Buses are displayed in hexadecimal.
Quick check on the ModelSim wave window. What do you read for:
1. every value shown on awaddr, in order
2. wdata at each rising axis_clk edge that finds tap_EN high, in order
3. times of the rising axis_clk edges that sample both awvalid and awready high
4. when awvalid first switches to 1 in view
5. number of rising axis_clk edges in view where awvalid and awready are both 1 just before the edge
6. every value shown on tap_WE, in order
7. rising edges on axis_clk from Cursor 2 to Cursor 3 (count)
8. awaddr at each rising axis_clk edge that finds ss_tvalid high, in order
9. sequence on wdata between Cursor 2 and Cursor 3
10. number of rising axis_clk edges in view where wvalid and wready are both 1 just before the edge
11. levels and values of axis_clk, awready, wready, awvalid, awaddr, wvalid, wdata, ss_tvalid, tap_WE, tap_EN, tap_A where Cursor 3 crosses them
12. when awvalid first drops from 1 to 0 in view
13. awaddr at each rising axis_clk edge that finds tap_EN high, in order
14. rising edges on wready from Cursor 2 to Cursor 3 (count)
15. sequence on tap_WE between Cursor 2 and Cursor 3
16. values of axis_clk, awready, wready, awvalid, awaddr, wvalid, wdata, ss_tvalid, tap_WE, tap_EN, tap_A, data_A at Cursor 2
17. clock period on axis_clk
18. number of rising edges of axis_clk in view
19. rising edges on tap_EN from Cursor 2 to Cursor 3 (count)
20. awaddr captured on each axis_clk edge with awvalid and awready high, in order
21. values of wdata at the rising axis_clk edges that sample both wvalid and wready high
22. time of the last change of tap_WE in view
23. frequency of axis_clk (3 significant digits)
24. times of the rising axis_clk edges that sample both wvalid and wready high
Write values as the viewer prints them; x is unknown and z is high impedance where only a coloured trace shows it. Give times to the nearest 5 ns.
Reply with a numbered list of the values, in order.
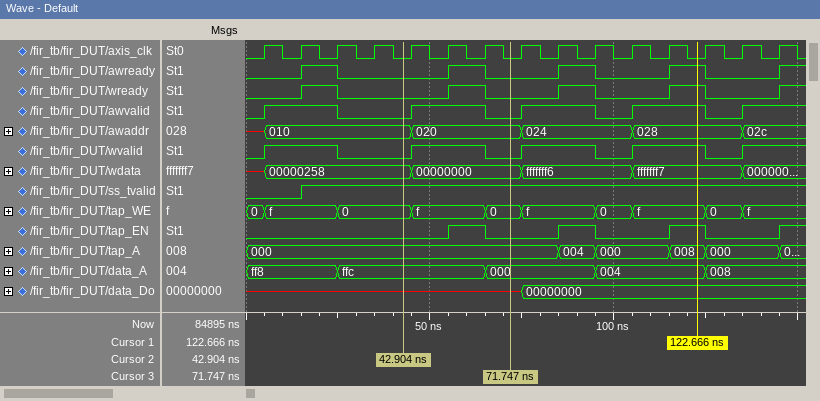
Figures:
1. x, 010, 020, 024, 028, 02c
2. 00000000, fffffff6, fffffff7
3. 25 ns, 65 ns, 95 ns, 125 ns
4. 5 ns
5. 4
6. 0, f, 0, f, 0, f, 0, f, 0, f
7. 3
8. 010, 010, 010, 020, 020, 020, 024, 024, 024, 028, 028, 028, 02c
9. 00000258, 00000000
10. 4
11. axis_clk=0, awready=0, wready=0, awvalid=0, awaddr=020, wvalid=0, wdata=00000000, ss_tvalid=1, tap_WE=0, tap_EN=0, tap_A=000
12. 25 ns
13. 020, 024, 028
14. 1
15. 0, f, 0
16. axis_clk=0, awready=0, wready=0, awvalid=0, awaddr=010, wvalid=0, wdata=00000258, ss_tvalid=1, tap_WE=0, tap_EN=0, tap_A=000, data_A=ffc
17. 10 ns
18. 15
19. 1
20. 010, 020, 024, 028
21. 00000258, 00000000, fffffff6, fffffff7
22. 135 ns
23. 100 MHz
24. 25 ns, 65 ns, 95 ns, 125 ns
